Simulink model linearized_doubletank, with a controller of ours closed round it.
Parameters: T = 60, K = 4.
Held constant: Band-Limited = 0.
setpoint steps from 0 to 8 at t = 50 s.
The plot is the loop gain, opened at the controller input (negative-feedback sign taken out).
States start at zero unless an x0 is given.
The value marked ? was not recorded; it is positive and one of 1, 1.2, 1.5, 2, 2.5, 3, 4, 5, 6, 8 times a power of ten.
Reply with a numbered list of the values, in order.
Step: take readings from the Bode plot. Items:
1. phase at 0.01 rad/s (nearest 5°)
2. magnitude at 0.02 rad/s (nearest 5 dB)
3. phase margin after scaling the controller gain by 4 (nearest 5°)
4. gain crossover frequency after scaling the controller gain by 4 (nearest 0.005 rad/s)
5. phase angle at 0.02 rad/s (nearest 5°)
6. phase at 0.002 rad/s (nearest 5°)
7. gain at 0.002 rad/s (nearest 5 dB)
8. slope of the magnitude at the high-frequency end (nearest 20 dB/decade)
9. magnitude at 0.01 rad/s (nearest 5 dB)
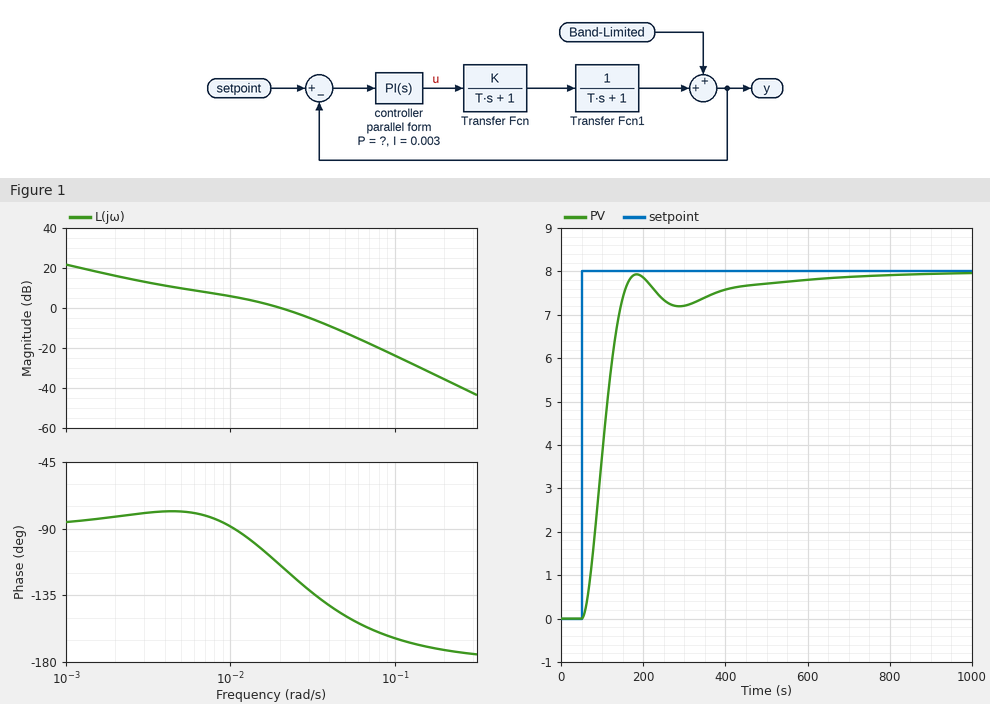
1. -90°
2. 0 dB
3. 30°
4. 0.050 rad/s
5. -115°
6. -80°
7. 15 dB
8. -40 dB/decade
9. 5 dB
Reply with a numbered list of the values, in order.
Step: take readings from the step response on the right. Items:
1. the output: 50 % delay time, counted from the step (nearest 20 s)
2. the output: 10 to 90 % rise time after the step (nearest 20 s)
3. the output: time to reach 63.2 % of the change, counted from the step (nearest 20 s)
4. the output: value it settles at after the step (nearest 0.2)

1. 60 s
2. 80 s
3. 60 s
4. 8.0
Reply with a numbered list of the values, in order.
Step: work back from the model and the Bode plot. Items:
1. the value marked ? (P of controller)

1. 0.6
